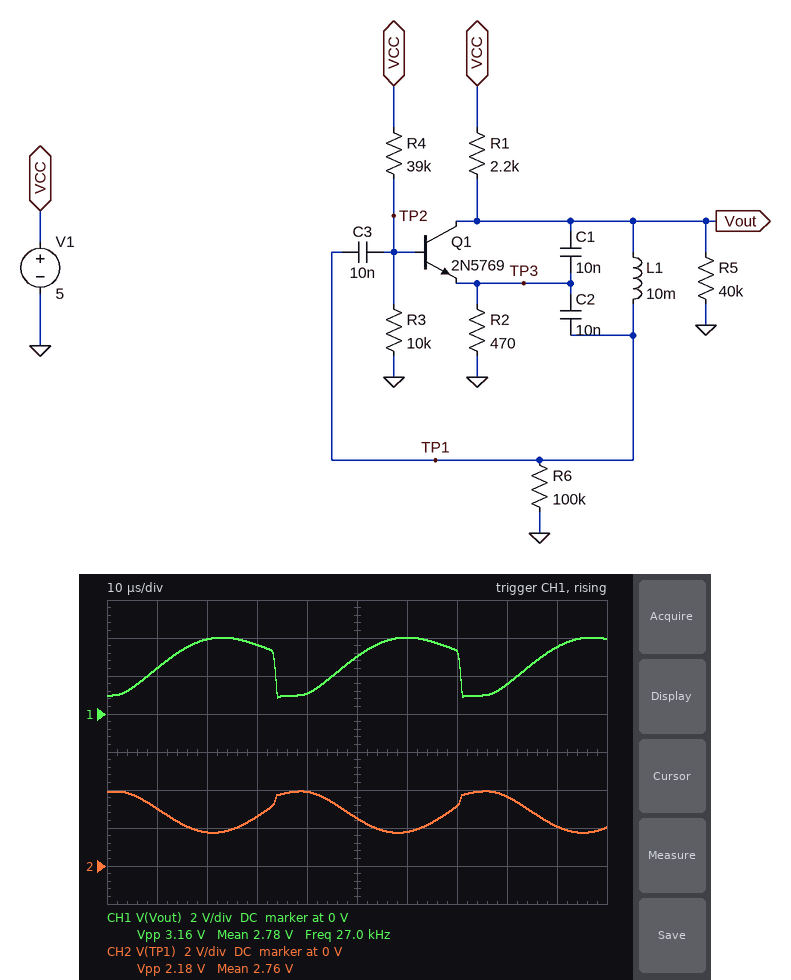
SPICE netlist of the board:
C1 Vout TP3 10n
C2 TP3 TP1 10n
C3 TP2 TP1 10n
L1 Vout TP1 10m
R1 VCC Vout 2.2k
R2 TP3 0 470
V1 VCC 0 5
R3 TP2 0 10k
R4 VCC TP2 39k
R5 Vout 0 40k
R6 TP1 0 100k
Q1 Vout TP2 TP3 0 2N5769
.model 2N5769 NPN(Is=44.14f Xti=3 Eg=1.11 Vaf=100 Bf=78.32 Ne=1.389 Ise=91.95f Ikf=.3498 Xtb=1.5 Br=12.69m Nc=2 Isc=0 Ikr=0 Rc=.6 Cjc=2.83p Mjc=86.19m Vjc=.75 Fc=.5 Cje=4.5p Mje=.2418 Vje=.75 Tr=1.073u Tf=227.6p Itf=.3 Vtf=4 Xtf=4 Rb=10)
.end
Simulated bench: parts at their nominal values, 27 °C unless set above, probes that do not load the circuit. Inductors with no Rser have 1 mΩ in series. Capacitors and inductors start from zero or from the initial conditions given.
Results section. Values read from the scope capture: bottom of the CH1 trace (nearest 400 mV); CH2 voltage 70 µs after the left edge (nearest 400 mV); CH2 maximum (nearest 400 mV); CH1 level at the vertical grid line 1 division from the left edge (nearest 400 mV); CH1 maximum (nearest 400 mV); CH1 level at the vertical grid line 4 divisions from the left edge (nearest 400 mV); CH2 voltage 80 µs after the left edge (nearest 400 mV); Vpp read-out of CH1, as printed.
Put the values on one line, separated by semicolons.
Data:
800 mV; 3.2 V; 4.0 V; 2.4 V; 4.0 V; 1.2 V; 3.6 V; 3.16 V
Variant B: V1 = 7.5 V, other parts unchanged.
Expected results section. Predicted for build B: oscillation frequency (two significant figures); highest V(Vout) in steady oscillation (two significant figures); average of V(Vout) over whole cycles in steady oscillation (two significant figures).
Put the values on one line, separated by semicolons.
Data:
28 kHz; 5.7 V; 3.9 V
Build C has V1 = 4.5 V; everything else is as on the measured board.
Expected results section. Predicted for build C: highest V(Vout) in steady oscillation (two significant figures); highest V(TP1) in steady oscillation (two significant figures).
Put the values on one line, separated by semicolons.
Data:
3.7 V; 3.6 V
